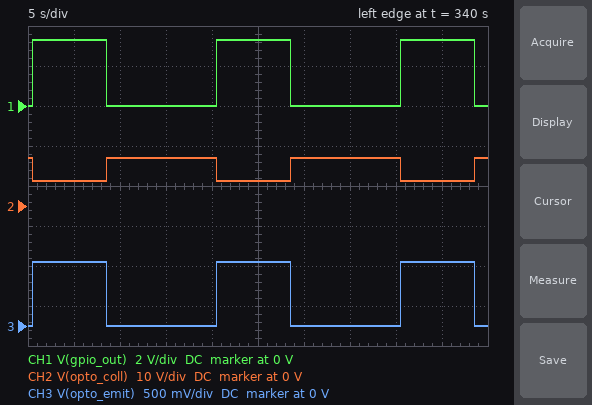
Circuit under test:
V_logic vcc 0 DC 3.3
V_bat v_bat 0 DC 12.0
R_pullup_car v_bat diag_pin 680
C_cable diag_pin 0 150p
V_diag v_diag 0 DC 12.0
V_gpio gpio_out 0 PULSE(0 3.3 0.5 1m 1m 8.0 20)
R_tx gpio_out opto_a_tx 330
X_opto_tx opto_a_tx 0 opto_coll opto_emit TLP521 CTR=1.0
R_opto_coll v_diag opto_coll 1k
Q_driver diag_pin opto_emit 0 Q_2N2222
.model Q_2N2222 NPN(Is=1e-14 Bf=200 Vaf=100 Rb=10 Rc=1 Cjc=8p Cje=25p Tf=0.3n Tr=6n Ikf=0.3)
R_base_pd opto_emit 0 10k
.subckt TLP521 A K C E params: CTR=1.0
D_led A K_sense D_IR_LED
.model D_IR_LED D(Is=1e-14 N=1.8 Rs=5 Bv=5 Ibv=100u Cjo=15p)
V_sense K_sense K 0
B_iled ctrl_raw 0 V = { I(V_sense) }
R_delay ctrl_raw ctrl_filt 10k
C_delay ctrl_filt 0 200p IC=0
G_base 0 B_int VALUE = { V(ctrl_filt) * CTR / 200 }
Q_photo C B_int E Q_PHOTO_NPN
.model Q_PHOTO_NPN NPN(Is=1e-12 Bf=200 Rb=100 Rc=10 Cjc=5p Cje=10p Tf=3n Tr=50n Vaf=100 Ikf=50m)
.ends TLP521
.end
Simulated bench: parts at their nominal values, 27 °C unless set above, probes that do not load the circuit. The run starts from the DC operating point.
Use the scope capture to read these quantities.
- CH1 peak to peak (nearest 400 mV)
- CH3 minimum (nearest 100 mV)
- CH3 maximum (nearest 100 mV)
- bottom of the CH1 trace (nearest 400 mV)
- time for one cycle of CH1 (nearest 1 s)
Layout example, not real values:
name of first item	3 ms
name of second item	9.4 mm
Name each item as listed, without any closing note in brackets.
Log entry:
CH1 peak to peak	3.2 V
CH3 minimum	0 V
CH3 maximum	800 mV
bottom of the CH1 trace	0 V
time for one cycle of CH1	20 s
